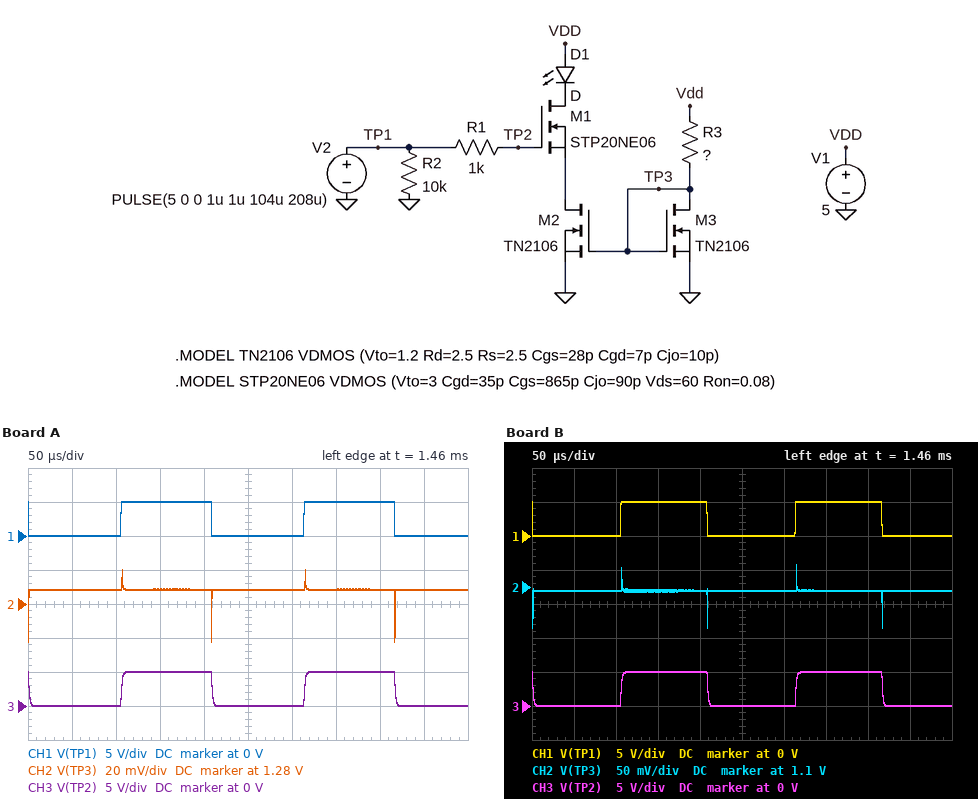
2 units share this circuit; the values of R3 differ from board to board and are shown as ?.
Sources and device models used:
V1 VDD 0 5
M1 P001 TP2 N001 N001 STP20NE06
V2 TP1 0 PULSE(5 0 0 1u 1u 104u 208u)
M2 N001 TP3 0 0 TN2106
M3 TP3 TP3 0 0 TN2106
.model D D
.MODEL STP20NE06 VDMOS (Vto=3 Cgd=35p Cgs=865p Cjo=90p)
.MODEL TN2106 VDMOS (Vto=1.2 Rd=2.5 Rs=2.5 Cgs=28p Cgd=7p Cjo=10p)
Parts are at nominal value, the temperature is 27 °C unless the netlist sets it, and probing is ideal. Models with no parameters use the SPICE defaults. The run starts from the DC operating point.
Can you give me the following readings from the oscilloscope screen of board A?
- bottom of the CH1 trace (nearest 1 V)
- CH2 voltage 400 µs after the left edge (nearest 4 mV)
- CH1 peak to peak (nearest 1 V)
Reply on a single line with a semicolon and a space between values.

0 V; 1.288 V; 5 V
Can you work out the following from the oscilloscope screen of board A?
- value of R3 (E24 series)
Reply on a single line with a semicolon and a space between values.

75 Ω
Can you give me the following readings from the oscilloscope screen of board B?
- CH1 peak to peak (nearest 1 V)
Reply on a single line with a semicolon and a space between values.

5 V
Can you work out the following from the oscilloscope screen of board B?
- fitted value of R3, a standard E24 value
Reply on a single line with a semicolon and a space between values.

390 Ω
